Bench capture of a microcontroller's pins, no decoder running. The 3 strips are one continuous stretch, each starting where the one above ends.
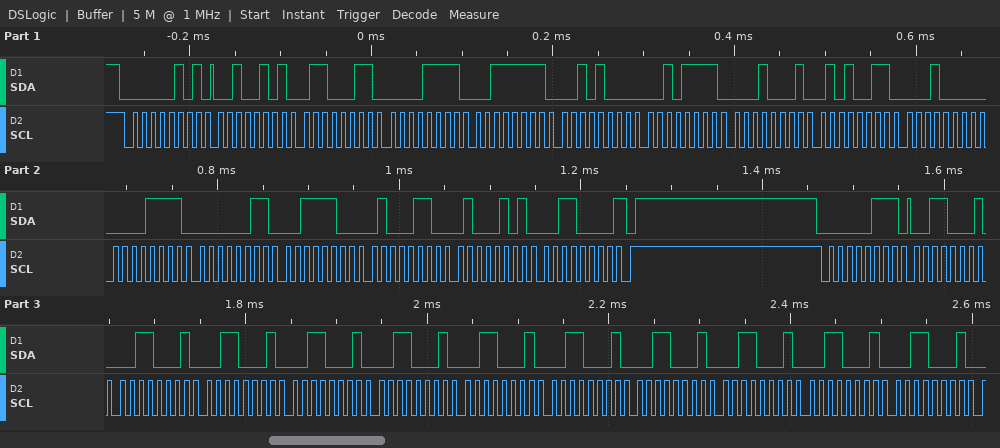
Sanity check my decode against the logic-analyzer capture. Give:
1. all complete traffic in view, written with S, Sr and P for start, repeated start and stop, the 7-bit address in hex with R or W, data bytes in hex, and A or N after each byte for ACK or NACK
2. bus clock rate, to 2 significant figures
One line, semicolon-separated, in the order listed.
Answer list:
S 02R A 25 A 63 A 0F A 3F A 28 A 2F A 11 A 53 A 10 A 0F A 03 A 3C A 46 A 45 A 30 N P S 03R A 31 A 31 A 31 A 31 A 31 A 31 A 31 A 31 A 31 A 31 A 31 A; 100 kHz
